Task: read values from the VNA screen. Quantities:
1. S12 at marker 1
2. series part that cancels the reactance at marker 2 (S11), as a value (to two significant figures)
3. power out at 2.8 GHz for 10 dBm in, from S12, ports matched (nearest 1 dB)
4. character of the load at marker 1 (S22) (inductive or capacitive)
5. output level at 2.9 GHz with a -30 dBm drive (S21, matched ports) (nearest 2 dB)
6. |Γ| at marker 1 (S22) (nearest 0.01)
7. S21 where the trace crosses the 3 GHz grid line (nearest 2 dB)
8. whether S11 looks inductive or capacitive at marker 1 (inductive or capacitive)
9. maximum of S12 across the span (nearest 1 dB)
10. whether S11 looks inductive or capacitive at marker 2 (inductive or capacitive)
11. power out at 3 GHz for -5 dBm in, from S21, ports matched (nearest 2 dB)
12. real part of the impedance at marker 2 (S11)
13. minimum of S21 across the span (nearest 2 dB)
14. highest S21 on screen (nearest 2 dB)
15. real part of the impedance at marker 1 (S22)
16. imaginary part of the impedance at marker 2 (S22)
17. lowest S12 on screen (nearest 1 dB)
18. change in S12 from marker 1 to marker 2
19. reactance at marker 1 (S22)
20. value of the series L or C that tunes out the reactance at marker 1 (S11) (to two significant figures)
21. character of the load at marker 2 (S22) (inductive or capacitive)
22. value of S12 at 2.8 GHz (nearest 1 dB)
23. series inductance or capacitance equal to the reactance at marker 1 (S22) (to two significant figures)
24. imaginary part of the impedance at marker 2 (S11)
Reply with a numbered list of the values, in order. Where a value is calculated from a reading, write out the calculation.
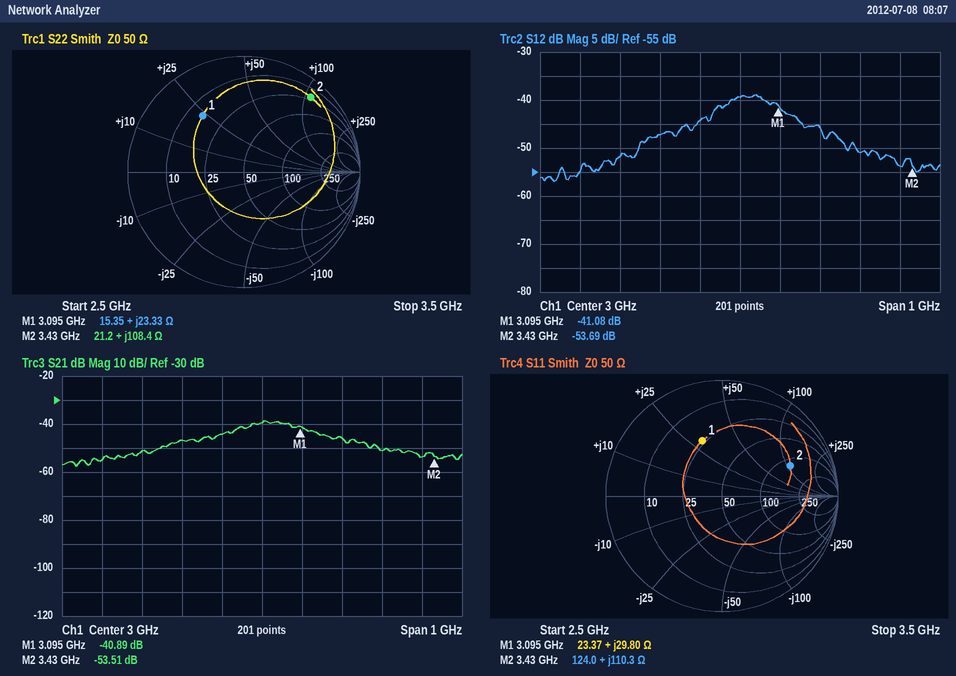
1. -41.08 dB
2. C = 1/(2π × 3.43 GHz × 110.3 Ω) ≈ 421 fF, so 420 fF to two significant figures
3. 10 dBm + (-47 dB) = -37 dBm
4. inductive
5. -30 dBm + (-44 dB) = -74 dBm
6. 0.60
7. -40 dB
8. inductive
9. -39 dB
10. inductive
11. -5 dBm + (-40 dB) = -44 dBm
12. 124.0 Ω
13. -58 dB
14. -38 dB
15. 15.35 Ω
16. +108.4 Ω
17. -57 dB
18. -53.69 − (-41.08) = -12.61 dB
19. +23.33 Ω
20. C = 1/(2π × 3.095 GHz × 29.8 Ω) ≈ 1.7 pF
21. inductive
22. -47 dB
23. L = 23.33 Ω/(2π × 3.095 GHz) ≈ 1.2 nH
24. +110.3 Ω
